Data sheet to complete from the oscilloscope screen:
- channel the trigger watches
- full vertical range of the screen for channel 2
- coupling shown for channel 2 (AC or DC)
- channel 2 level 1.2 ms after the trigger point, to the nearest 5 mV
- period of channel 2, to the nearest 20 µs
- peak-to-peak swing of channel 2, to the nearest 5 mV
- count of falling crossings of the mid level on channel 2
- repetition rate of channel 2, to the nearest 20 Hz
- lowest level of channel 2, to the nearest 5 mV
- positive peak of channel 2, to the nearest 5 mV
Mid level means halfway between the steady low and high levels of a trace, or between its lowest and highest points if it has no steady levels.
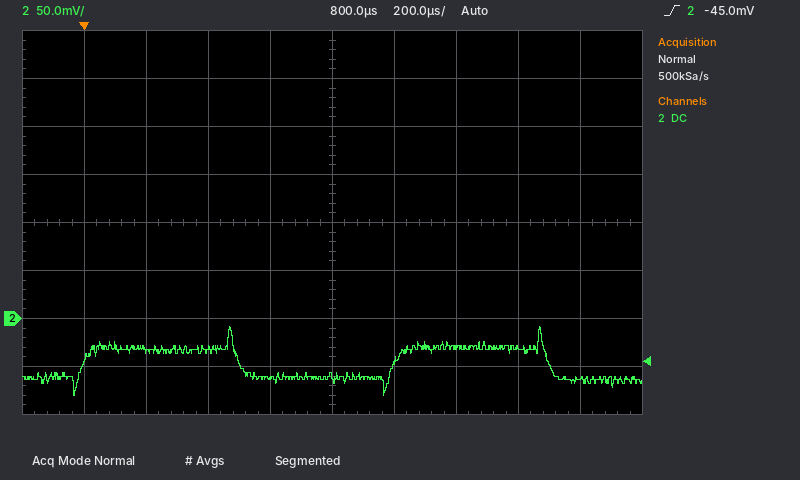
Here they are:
channel 2
400 mV
DC
-30 mV
1.00 ms
70 mV
2
1.00 kHz
-80 mV
-10 mV
